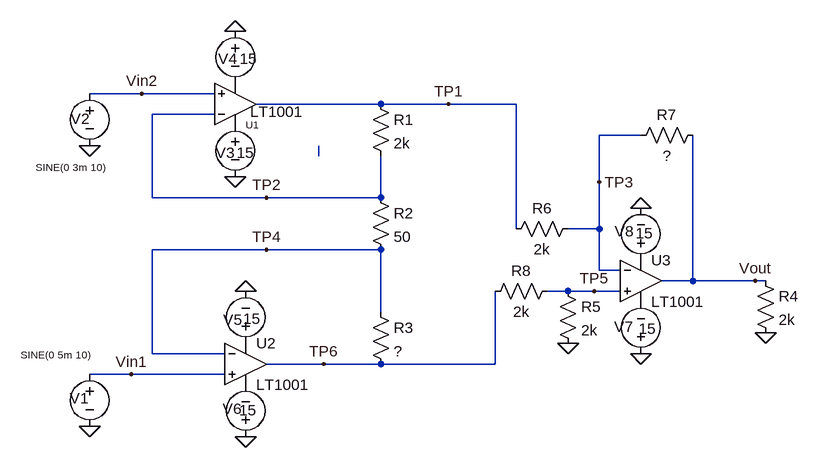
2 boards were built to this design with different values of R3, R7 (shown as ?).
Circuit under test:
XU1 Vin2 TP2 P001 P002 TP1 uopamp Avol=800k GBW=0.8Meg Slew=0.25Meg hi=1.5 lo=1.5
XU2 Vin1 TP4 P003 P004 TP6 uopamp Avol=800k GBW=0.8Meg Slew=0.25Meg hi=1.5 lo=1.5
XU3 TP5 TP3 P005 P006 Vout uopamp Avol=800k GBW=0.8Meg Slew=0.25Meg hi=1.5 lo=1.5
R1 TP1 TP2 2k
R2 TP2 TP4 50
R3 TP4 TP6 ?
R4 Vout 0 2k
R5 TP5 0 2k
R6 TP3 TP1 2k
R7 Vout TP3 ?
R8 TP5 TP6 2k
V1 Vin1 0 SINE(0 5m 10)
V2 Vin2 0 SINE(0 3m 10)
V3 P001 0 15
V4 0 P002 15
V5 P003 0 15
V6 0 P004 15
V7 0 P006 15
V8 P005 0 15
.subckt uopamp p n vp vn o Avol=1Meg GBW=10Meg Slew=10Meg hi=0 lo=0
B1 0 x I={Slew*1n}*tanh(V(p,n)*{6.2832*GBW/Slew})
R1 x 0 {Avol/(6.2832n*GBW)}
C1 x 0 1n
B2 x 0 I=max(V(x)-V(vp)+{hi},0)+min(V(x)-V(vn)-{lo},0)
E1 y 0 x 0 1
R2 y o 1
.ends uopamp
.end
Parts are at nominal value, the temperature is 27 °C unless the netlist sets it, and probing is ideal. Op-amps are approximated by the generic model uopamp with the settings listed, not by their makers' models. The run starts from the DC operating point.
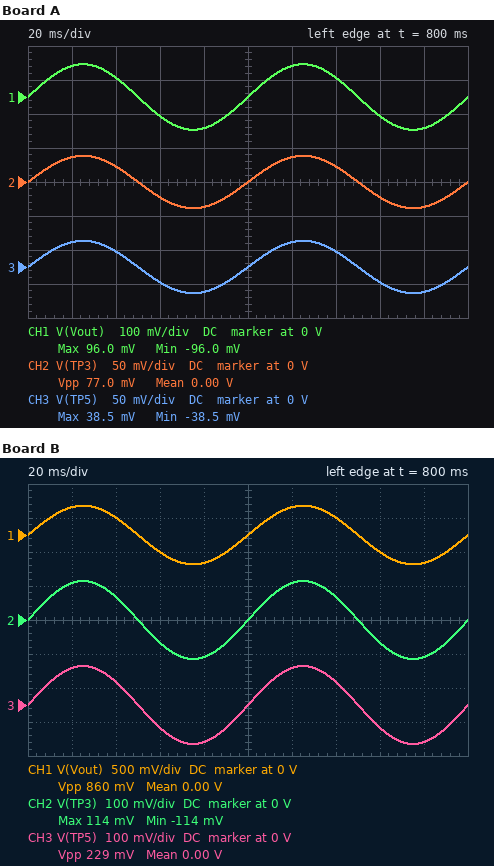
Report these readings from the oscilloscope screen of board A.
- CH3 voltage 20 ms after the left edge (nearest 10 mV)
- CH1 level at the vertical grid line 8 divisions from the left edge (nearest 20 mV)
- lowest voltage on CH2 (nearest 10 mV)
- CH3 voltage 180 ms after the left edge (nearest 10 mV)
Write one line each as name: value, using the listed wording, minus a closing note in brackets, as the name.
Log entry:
CH3 voltage 20 ms after the left edge: 40 mV
CH1 level at the vertical grid line 8 divisions from the left edge: -60 mV
lowest voltage on CH2: -40 mV
CH3 voltage 180 ms after the left edge: -40 mV
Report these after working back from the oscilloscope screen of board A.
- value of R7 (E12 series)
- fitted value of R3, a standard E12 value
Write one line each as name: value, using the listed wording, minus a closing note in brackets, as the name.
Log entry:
value of R7: 1 kΩ
fitted value of R3, a standard E12 value: 1.8 kΩ
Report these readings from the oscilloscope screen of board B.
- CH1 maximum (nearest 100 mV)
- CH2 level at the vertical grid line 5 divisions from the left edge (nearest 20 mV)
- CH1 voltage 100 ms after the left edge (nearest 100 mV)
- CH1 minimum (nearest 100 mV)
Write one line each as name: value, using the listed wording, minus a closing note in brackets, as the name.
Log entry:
CH1 maximum: 400 mV
CH2 level at the vertical grid line 5 divisions from the left edge: 0 V
CH1 voltage 100 ms after the left edge: 0 V
CH1 minimum: -400 mV
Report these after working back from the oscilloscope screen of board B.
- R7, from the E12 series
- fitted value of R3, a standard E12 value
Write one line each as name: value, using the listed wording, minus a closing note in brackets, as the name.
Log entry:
R7, from the E12 series: 3.3 kΩ
fitted value of R3, a standard E12 value: 5.6 kΩ
